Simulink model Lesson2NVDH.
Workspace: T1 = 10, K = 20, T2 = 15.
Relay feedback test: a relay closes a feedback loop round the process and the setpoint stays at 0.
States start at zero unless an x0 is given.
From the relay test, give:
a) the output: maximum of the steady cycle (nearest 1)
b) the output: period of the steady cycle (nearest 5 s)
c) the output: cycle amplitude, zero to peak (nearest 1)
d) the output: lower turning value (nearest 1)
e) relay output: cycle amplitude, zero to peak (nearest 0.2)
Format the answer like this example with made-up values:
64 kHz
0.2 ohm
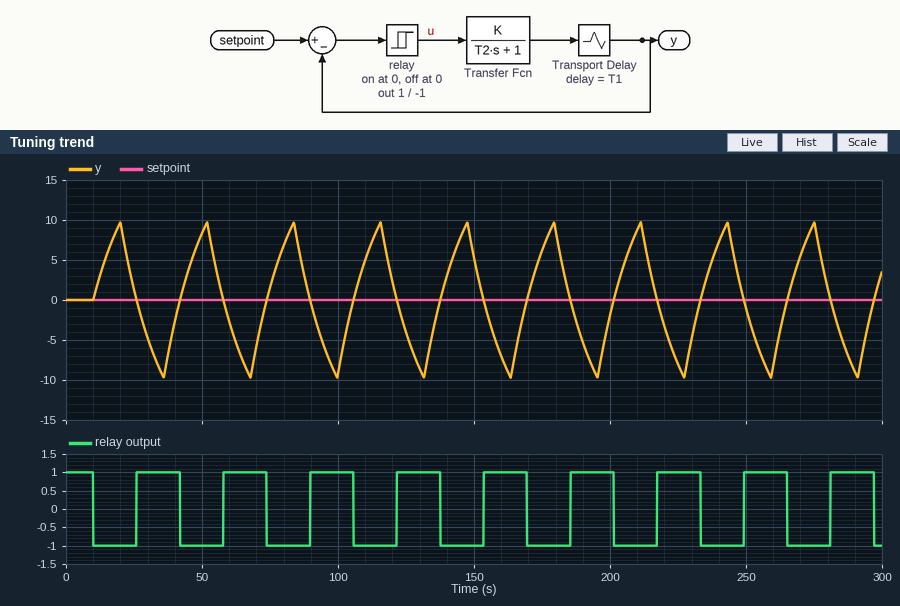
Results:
10
30 s
10
-10
1.0
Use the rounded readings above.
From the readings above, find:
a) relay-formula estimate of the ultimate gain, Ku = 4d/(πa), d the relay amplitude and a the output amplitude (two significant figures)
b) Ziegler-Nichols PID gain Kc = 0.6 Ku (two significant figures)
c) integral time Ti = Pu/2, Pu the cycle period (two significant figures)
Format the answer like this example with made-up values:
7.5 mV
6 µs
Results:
0.13
0.078
15 s
